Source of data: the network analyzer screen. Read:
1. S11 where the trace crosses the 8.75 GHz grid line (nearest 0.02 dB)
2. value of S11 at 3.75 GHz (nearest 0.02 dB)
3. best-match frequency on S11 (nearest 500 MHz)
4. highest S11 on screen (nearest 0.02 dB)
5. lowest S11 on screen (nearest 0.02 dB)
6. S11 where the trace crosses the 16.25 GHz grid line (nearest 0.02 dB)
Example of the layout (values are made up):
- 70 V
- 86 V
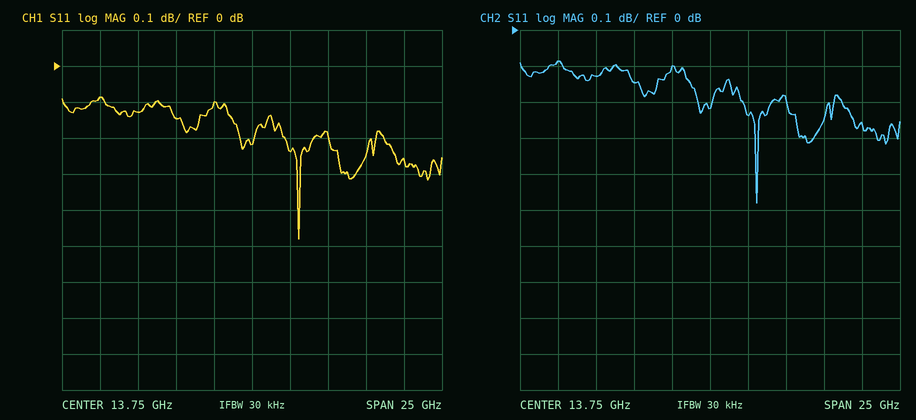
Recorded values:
- -0.14 dB
- -0.08 dB
- 17.0 GHz
- -0.08 dB
- -0.48 dB
- -0.24 dB
